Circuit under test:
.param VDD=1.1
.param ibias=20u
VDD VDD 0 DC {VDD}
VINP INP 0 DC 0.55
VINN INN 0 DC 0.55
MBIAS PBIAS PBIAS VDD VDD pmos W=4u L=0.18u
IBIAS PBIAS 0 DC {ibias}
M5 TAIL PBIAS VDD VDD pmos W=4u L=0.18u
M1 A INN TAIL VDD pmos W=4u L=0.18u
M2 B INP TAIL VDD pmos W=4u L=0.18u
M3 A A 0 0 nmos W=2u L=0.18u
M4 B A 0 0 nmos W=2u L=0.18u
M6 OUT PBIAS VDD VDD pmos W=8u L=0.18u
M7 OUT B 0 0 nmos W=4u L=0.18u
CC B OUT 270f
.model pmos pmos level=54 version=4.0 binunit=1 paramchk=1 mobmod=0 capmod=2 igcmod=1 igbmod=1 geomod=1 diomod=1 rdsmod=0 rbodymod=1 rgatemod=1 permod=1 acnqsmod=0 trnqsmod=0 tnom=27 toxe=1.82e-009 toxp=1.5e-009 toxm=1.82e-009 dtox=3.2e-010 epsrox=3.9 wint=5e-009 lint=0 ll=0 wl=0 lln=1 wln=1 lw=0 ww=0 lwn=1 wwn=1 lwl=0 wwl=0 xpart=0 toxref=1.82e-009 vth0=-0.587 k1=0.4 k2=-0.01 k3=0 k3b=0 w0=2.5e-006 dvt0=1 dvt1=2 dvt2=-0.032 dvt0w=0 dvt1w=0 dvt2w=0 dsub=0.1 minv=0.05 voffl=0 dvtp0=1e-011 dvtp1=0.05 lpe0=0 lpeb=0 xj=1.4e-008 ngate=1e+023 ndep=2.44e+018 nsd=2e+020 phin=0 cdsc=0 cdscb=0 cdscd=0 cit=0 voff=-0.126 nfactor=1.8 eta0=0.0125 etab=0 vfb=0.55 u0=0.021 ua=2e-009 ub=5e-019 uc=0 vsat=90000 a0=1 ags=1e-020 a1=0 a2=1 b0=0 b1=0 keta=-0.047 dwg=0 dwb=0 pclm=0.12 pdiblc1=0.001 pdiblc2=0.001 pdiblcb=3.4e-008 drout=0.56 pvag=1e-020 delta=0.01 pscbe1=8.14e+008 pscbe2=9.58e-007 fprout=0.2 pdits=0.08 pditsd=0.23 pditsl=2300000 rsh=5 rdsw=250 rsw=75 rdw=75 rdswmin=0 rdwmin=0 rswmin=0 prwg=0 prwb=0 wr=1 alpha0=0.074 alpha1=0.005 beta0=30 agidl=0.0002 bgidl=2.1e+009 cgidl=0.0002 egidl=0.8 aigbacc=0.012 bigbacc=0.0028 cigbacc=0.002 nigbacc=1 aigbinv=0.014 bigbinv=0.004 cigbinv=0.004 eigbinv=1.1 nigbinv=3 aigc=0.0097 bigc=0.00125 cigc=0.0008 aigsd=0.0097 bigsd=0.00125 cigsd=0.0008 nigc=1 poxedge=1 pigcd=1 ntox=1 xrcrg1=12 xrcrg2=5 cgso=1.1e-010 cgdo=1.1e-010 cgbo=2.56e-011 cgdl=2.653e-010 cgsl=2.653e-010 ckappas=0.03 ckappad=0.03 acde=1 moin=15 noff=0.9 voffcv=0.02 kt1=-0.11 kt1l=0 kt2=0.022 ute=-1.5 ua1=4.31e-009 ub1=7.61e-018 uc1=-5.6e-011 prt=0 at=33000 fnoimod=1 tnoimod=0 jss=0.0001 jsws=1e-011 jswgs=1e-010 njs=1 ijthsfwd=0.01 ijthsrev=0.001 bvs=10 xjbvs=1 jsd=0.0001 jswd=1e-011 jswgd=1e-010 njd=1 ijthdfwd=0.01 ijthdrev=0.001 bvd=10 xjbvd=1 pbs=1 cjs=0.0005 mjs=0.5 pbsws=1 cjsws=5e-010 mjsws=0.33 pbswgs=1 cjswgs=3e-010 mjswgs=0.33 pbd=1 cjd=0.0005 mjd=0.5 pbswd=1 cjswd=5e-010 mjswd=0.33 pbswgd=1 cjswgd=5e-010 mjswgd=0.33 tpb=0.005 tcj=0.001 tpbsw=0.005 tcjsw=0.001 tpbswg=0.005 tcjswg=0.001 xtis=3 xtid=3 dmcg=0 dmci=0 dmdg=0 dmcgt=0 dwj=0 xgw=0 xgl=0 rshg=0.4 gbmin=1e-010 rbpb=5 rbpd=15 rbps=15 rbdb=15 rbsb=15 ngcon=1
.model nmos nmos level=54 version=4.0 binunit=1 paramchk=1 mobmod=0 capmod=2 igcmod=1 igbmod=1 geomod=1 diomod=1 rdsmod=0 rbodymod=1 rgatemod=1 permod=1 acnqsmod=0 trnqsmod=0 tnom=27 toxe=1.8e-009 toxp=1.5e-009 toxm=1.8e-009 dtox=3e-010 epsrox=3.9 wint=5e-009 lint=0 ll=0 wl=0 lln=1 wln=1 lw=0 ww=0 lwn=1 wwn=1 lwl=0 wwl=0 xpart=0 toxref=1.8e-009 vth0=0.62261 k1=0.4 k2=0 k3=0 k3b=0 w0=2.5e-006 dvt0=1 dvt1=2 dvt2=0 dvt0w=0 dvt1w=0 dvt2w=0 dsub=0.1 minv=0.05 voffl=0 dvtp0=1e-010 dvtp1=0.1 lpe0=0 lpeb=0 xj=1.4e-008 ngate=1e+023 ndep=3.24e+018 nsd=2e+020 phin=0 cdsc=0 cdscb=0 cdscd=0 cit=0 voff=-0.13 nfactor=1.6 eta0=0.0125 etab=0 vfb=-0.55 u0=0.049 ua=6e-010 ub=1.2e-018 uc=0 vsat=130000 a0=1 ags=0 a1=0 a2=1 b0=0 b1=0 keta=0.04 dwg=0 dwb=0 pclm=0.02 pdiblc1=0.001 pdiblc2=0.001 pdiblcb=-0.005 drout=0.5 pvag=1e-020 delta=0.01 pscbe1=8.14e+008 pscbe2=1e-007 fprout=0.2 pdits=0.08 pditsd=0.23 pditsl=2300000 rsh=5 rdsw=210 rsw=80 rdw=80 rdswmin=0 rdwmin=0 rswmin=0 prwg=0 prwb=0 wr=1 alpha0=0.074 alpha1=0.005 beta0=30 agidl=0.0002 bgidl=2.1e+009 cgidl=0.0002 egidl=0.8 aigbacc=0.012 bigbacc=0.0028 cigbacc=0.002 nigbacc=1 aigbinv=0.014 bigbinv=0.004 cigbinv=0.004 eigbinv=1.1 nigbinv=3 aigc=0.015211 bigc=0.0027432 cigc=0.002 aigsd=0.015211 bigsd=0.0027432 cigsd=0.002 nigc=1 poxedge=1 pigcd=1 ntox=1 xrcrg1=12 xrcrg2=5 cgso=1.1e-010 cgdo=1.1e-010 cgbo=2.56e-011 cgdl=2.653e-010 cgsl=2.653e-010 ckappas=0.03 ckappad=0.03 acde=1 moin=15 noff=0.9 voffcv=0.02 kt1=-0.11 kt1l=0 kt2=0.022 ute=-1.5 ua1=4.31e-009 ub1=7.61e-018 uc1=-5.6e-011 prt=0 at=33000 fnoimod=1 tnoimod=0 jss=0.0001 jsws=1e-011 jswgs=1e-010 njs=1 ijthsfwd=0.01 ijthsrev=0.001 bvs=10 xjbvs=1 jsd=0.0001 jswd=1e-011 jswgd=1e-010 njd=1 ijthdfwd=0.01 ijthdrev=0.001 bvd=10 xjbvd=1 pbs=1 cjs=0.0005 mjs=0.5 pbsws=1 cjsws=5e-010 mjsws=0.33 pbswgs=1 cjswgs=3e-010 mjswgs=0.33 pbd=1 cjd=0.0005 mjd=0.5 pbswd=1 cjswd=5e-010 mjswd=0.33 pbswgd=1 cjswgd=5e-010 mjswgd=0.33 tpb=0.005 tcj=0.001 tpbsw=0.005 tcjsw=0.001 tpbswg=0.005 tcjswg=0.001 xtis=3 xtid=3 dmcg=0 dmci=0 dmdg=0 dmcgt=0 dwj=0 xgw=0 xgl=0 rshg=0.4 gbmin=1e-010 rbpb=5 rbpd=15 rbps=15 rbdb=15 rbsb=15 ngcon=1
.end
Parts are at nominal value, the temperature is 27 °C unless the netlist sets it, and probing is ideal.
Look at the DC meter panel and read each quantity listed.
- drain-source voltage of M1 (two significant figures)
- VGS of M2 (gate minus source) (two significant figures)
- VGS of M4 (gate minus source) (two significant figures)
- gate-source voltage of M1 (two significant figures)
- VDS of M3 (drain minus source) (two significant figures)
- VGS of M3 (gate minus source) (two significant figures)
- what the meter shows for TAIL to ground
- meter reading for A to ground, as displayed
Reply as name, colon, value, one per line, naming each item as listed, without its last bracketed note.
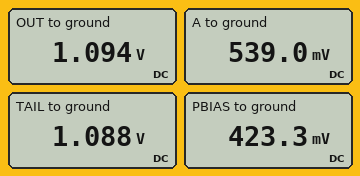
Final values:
drain-source voltage of M1: -550 mV
VGS of M2 (gate minus source): -540 mV
VGS of M4 (gate minus source): 540 mV
gate-source voltage of M1: -540 mV
VDS of M3 (drain minus source): 540 mV
VGS of M3 (gate minus source): 540 mV
what the meter shows for TAIL to ground: 1.088 V
meter reading for A to ground, as displayed: 539.0 mV
